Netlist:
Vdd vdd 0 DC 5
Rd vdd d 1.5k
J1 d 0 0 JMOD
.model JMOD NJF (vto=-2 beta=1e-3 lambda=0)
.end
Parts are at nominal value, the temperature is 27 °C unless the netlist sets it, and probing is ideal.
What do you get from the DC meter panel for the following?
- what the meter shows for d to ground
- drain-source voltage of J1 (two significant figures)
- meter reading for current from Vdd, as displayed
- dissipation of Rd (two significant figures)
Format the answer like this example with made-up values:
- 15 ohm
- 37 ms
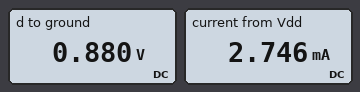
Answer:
- 0.880 V
- 880 mV
- 2.746 mA
- 11 mW
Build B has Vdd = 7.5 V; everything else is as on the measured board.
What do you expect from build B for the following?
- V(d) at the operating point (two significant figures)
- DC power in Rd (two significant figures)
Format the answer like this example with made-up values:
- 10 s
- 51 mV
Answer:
- 1.7 V
- 23 mW
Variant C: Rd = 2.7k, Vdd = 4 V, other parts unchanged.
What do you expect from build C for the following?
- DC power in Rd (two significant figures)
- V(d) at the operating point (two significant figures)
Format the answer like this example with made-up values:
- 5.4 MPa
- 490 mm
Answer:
- 4.9 mW
- 370 mV
